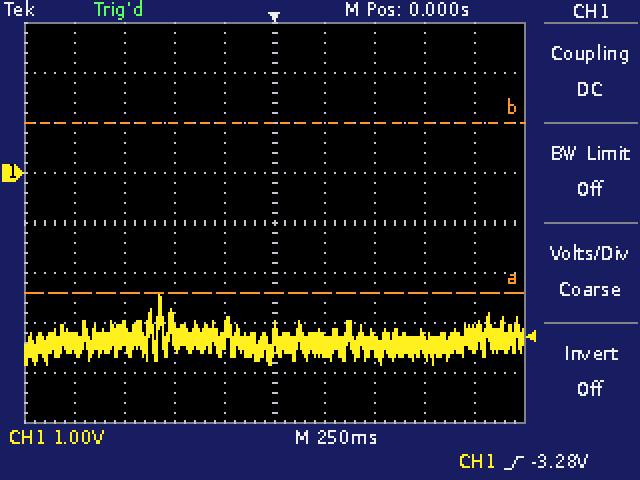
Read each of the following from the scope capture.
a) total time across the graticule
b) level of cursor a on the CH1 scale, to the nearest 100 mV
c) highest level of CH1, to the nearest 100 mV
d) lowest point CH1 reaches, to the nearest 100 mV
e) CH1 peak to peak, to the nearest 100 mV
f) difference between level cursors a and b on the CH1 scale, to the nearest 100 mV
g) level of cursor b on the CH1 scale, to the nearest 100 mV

2.5 s
-2.4 V
-2.4 V
-3.8 V
1.4 V
3.4 V
1.0 V
